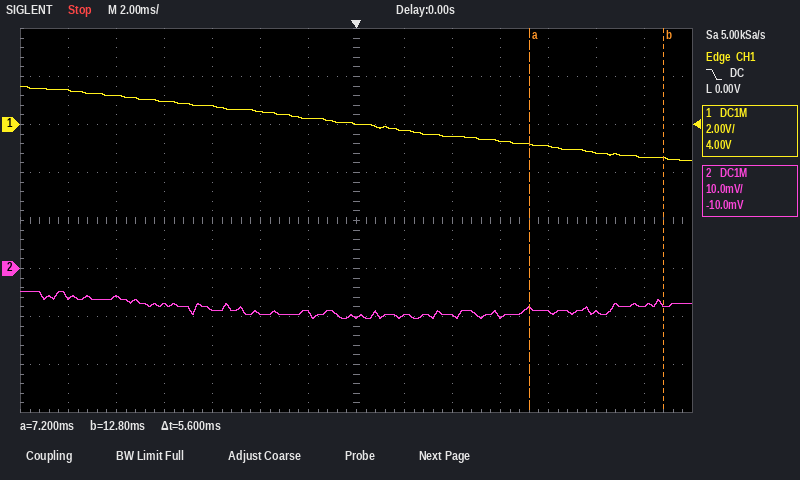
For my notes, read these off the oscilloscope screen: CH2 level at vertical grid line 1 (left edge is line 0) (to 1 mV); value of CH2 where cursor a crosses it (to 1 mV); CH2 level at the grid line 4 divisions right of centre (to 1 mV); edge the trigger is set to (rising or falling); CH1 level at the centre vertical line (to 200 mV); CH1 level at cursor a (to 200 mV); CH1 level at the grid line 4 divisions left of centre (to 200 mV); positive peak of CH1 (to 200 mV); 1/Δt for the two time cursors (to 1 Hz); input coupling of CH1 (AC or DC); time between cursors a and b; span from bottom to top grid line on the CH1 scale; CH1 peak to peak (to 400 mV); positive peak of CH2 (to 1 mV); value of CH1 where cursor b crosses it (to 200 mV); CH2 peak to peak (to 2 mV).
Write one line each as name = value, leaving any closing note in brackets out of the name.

CH2 level at vertical grid line 1 (left edge is line 0) = -6 mV
value of CH2 where cursor a crosses it = -8 mV
CH2 level at the grid line 4 divisions right of centre = -9 mV
edge the trigger is set to = falling
CH1 level at the centre vertical line = 0.0 V
CH1 level at cursor a = -800 mV
CH1 level at the grid line 4 divisions left of centre = 1.0 V
positive peak of CH1 = 1.6 V
1/Δt for the two time cursors = 179 Hz
input coupling of CH1 = DC
time between cursors a and b = 5.6 ms
span from bottom to top grid line on the CH1 scale = 16 V
CH1 peak to peak = 3.2 V
positive peak of CH2 = -5 mV
value of CH1 where cursor b crosses it = -1.4 V
CH2 peak to peak = 6 mV
